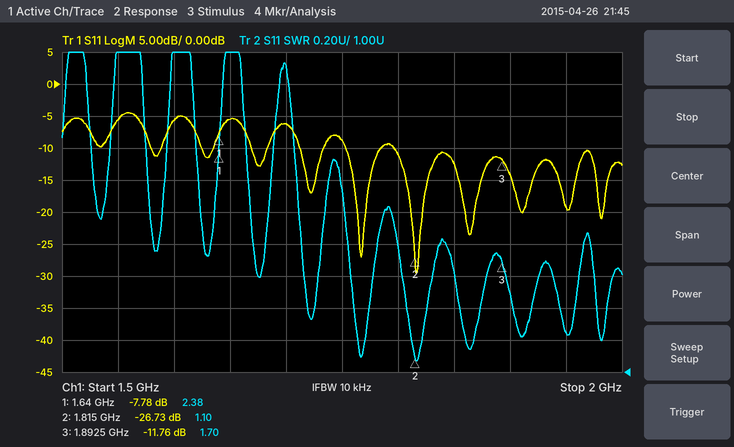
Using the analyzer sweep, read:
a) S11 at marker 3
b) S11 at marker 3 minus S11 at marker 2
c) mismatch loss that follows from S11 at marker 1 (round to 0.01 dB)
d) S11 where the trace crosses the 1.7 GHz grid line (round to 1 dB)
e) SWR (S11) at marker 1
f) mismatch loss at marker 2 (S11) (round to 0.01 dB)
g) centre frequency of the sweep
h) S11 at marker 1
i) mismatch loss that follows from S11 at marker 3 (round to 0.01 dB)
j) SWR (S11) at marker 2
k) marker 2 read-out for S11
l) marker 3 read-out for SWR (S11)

-11.76 dB
14.97 dB
0.79 dB
-6 dB
2.38
0.01 dB
1.75 GHz
-7.78 dB
0.30 dB
1.10
-26.73 dB
1.70
